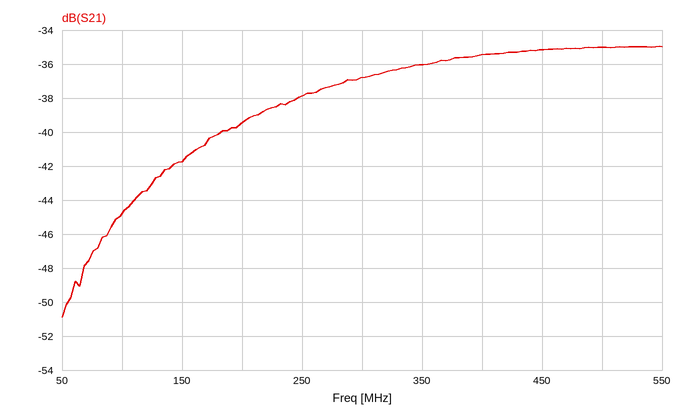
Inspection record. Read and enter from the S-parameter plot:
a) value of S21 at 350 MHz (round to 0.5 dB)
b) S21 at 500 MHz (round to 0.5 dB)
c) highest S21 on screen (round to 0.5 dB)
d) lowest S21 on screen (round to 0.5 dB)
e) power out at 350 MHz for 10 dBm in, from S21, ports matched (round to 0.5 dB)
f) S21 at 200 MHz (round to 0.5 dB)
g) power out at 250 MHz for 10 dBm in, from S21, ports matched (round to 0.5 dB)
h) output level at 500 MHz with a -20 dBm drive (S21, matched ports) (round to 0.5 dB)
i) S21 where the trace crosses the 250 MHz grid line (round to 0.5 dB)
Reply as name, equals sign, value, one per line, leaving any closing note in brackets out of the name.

value of S21 at 350 MHz = -36.0 dB
S21 at 500 MHz = -35.0 dB
highest S21 on screen = -35.0 dB
lowest S21 on screen = -51.0 dB
power out at 350 MHz for 10 dBm in, from S21, ports matched = -26.0 dBm
S21 at 200 MHz = -39.5 dB
power out at 250 MHz for 10 dBm in, from S21, ports matched = -28.0 dBm
output level at 500 MHz with a -20 dBm drive (S21, matched ports) = -55.0 dBm
S21 where the trace crosses the 250 MHz grid line = -38.0 dB
